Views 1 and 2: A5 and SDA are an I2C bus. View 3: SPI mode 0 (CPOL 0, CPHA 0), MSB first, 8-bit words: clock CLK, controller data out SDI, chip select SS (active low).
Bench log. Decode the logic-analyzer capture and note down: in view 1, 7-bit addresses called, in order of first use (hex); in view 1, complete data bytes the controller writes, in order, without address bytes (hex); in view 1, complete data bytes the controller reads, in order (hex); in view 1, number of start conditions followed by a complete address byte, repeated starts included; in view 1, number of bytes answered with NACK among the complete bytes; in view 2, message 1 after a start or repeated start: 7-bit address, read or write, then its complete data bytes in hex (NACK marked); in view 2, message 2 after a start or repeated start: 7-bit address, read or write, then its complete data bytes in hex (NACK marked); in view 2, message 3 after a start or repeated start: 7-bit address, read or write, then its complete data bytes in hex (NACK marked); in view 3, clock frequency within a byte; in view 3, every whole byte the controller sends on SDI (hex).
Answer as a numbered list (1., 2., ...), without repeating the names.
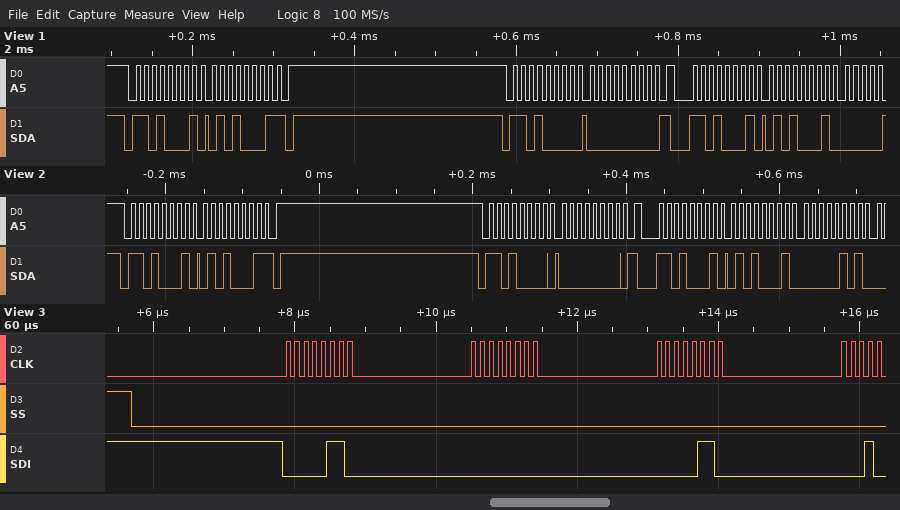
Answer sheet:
1. 0x68
2. 00
3. 51 51
4. 3
5. 1
6. 0x68 read: 51 NACK
7. 0x68 write: 00
8. 0x68 read: 51 05
9. 8 MHz
10. 06 00 06
